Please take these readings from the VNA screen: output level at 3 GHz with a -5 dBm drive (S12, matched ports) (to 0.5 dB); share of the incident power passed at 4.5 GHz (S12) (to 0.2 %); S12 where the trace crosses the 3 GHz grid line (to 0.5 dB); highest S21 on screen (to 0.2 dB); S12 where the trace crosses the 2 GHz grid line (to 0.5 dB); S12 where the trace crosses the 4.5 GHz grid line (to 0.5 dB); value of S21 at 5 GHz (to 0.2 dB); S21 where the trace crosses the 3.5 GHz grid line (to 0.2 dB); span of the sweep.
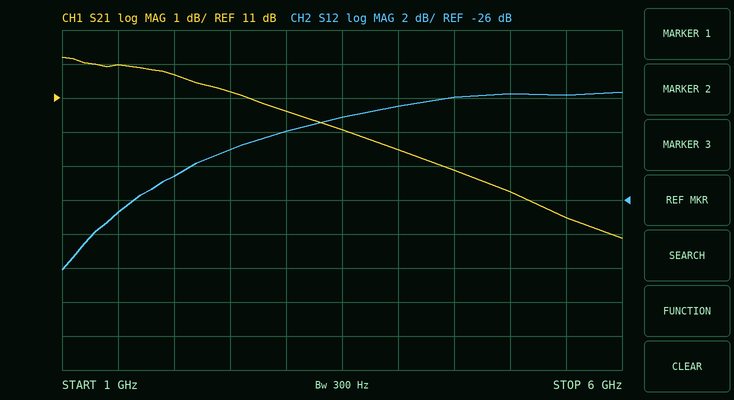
-27.0 dBm
1.0 %
-22.0 dB
12.2 dB
-24.5 dB
-20.0 dB
8.2 dB
10.0 dB
5 GHz
